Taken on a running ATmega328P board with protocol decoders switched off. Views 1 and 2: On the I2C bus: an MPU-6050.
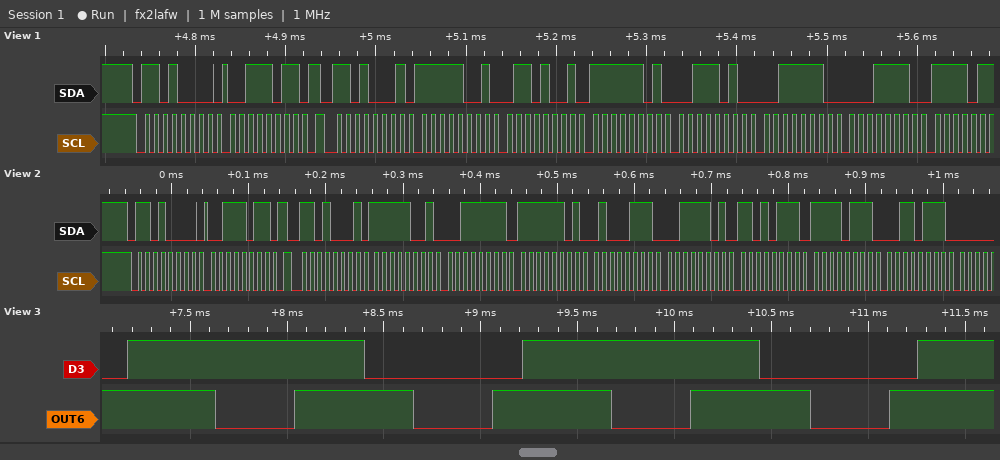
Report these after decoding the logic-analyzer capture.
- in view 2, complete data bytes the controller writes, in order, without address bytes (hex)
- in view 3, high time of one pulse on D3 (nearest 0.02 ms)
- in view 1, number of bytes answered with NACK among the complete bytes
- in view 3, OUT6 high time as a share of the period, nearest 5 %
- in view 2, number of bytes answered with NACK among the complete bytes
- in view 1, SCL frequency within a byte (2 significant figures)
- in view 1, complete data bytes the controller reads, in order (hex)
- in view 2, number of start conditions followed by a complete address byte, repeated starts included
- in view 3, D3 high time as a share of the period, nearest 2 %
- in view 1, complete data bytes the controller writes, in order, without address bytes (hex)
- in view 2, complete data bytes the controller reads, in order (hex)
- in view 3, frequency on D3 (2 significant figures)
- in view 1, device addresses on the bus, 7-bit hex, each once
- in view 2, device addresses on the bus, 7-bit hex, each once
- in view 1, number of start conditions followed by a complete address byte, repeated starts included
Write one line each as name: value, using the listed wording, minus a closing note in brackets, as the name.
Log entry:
in view 2, complete data bytes the controller writes, in order, without address bytes: 3B
in view 3, high time of one pulse on D3: 1.22 ms
in view 1, number of bytes answered with NACK among the complete bytes: 0
in view 3, OUT6 high time as a share of the period, nearest 5 %: 60 %
in view 2, number of bytes answered with NACK among the complete bytes: 0
in view 1, SCL frequency within a byte: 100 kHz
in view 1, complete data bytes the controller reads, in order: F9 69 FD 3A 3E 1E
in view 2, number of start conditions followed by a complete address byte, repeated starts included: 2
in view 3, D3 high time as a share of the period, nearest 2 %: 60 %
in view 1, complete data bytes the controller writes, in order, without address bytes: 3B
in view 2, complete data bytes the controller reads, in order: F9 3F FD 47 3D D7 F7 37
in view 3, frequency on D3: 490 Hz
in view 1, device addresses on the bus, 7-bit hex, each once: 0x68
in view 2, device addresses on the bus, 7-bit hex, each once: 0x68
in view 1, number of start conditions followed by a complete address byte, repeated starts included: 2
